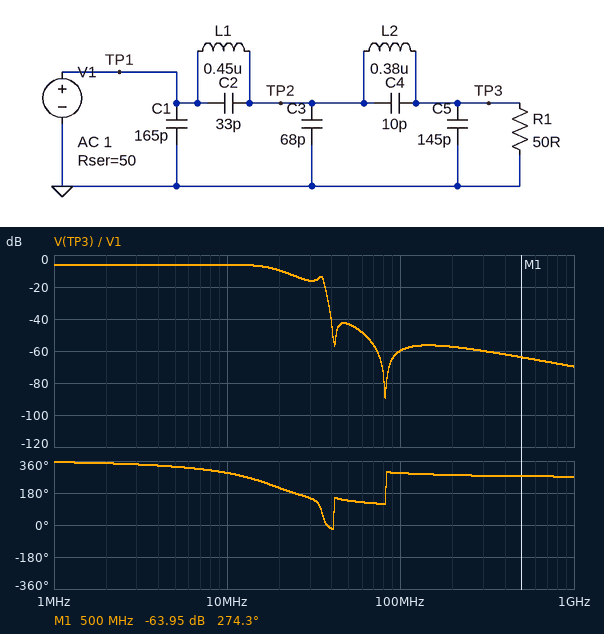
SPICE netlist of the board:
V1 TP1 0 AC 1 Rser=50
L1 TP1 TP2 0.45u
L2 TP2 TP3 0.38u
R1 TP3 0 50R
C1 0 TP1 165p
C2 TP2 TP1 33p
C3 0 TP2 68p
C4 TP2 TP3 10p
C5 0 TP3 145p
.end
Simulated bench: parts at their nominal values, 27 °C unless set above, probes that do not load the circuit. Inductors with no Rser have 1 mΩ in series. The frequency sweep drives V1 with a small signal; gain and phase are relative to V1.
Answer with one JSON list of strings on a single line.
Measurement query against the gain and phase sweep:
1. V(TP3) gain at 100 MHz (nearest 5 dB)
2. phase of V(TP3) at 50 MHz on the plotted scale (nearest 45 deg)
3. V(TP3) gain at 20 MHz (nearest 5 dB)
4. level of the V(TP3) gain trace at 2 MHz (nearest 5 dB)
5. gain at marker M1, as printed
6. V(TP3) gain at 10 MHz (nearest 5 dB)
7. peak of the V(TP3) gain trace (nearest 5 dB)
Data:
["-60 dB", "135 deg", "-10 dB", "-5 dB", "-63.95 dB", "-5 dB", "-5 dB"]
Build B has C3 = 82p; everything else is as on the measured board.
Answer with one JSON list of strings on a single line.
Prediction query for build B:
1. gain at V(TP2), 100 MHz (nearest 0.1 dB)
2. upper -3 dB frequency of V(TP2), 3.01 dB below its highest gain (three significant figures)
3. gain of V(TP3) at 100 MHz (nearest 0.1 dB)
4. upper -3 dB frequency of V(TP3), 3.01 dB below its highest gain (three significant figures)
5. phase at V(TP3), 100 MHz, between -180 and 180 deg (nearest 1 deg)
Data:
["-27.7 dB", "34.6 MHz", "-60.9 dB", "19.5 MHz", "-68 deg"]
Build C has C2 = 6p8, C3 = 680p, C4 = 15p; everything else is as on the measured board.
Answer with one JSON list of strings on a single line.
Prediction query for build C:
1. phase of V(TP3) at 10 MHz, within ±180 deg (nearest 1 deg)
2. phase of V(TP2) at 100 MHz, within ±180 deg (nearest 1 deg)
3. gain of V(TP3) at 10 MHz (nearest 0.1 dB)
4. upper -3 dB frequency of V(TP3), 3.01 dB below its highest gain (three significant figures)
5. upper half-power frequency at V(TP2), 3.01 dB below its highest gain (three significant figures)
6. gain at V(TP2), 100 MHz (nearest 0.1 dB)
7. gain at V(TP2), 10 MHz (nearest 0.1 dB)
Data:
["-107 deg", "-79 deg", "-7.8 dB", "17.4 MHz", "13.2 MHz", "-69.9 dB", "-8.6 dB"]
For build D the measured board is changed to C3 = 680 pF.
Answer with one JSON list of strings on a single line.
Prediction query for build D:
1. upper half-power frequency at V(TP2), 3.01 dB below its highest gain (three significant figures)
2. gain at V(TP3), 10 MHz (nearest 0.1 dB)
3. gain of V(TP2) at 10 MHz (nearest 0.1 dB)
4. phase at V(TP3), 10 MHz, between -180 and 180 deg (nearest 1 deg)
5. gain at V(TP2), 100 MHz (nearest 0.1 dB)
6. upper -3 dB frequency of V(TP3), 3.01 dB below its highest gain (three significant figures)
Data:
["12.9 MHz", "-7.8 dB", "-8.5 dB", "-108 deg", "-44.0 dB", "16.3 MHz"]
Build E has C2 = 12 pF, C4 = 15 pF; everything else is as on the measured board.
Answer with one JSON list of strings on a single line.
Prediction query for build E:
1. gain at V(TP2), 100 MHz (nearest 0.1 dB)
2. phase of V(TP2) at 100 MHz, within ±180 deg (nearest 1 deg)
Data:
["-37.0 dB", "-79 deg"]
